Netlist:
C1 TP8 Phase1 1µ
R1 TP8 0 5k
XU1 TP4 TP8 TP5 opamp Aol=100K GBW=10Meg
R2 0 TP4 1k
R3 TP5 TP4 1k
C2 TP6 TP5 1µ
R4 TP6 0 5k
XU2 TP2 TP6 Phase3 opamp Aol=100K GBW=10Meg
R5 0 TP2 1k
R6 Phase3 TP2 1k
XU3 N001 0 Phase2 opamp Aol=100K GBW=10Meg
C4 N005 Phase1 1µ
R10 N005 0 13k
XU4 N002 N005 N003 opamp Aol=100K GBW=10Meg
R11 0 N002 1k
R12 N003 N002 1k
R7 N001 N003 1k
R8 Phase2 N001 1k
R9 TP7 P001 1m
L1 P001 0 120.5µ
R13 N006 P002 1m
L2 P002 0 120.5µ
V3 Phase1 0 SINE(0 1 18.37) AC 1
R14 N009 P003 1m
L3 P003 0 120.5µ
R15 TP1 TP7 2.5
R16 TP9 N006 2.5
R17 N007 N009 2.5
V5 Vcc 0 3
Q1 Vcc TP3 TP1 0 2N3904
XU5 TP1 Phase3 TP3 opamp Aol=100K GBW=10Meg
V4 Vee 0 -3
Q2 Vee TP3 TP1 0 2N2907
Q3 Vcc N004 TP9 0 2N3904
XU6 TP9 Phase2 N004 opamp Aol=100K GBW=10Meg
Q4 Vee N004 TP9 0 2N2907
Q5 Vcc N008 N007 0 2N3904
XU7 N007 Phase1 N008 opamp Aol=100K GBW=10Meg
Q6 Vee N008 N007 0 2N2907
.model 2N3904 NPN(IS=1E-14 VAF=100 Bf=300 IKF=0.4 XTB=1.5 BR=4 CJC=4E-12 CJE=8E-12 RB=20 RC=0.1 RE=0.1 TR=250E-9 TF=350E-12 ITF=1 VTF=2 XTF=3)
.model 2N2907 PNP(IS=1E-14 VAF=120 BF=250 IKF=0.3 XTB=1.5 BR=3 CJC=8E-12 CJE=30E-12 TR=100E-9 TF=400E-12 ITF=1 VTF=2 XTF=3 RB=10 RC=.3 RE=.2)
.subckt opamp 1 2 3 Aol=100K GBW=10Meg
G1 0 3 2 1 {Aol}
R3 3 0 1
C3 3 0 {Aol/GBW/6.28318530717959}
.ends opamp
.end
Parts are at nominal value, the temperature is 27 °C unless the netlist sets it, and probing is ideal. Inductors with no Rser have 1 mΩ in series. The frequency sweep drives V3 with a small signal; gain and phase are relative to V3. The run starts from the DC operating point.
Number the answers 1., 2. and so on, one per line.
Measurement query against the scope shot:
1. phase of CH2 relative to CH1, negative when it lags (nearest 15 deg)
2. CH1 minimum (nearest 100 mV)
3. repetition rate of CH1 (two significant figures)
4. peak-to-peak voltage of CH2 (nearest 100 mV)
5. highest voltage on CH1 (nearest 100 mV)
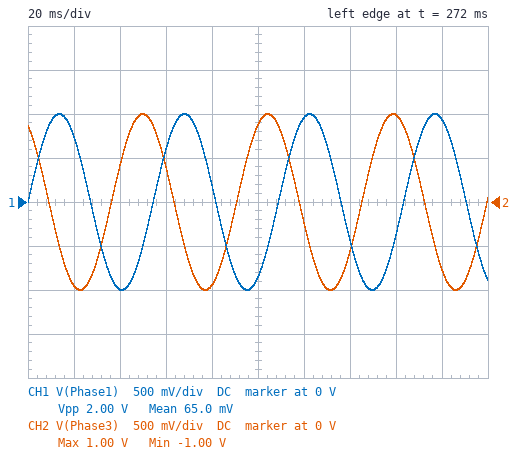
1. 120 deg
2. -1.0 V
3. 18 Hz
4. 2.0 V
5. 1.0 V
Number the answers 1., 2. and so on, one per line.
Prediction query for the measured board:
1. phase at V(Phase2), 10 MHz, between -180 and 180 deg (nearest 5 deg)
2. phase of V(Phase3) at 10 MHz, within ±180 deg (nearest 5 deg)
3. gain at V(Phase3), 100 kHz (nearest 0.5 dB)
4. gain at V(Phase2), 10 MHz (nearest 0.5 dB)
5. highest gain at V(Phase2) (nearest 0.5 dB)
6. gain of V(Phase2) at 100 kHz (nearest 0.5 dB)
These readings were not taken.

1. 55 deg
2. -125 deg
3. 12.0 dB
4. -8.0 dB
5. 6.0 dB
6. 6.0 dB
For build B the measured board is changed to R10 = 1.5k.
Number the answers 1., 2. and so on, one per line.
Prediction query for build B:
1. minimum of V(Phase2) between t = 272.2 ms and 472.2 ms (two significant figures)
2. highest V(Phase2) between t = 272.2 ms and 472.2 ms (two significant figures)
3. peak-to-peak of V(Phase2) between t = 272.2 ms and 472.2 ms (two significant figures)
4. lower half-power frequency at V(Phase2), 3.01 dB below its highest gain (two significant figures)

1. -340 mV
2. 340 mV
3. 680 mV
4. 110 Hz
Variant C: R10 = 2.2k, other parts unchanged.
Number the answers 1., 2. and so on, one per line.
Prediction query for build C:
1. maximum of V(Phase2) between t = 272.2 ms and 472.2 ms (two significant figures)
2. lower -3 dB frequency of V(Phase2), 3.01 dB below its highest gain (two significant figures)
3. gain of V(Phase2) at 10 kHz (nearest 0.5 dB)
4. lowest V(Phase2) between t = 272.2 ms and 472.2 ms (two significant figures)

1. 490 mV
2. 72 Hz
3. 6.0 dB
4. -490 mV
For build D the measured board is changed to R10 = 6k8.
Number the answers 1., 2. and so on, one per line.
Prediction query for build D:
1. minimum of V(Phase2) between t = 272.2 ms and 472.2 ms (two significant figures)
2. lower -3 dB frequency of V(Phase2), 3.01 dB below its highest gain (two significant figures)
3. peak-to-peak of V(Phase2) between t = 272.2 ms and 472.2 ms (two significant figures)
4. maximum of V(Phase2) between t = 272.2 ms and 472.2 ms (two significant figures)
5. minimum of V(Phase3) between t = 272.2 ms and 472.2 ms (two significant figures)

1. -1.2 V
2. 23 Hz
3. 2.5 V
4. 1.2 V
5. -1.0 V
